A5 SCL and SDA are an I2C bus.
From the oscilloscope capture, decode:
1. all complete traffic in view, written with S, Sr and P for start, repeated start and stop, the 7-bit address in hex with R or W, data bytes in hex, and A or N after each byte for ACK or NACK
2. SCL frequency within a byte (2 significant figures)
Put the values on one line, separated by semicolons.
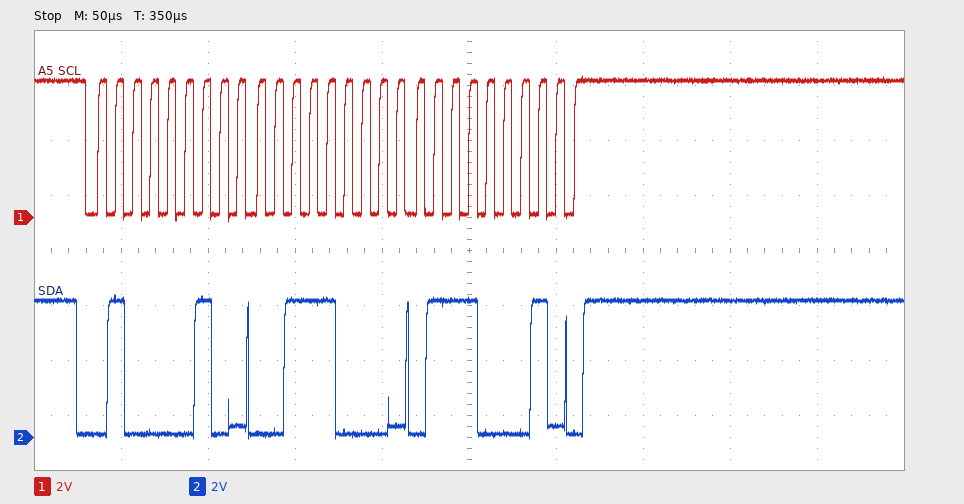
S 21W A 38 A 71 A P; 100 kHz
